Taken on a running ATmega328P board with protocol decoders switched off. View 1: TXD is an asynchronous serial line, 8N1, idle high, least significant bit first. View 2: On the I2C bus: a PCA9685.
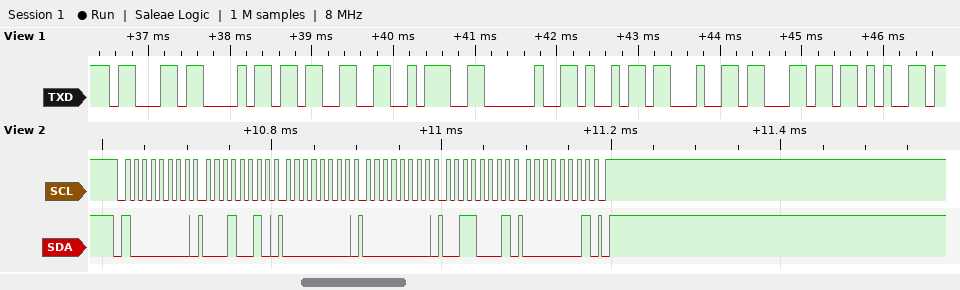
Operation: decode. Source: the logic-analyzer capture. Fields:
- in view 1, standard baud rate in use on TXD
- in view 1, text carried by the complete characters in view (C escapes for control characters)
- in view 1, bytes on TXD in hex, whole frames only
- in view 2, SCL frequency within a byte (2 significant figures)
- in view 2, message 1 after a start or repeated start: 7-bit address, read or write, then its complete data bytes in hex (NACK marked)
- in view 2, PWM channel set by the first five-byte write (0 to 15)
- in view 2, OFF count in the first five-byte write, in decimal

9600 baud
"ch3: idle"
63 68 33 3A 20 69 64 6C 65
100 kHz
0x40 write: 12 00 00 31 01
3
305
